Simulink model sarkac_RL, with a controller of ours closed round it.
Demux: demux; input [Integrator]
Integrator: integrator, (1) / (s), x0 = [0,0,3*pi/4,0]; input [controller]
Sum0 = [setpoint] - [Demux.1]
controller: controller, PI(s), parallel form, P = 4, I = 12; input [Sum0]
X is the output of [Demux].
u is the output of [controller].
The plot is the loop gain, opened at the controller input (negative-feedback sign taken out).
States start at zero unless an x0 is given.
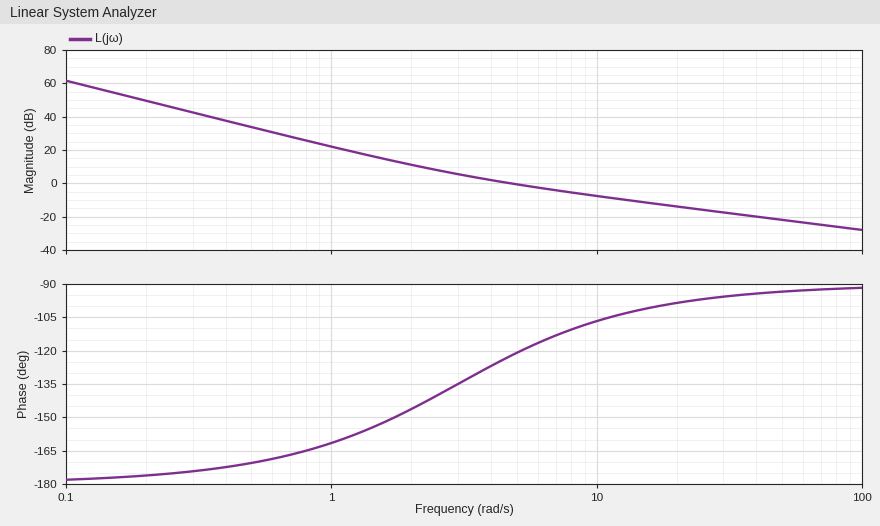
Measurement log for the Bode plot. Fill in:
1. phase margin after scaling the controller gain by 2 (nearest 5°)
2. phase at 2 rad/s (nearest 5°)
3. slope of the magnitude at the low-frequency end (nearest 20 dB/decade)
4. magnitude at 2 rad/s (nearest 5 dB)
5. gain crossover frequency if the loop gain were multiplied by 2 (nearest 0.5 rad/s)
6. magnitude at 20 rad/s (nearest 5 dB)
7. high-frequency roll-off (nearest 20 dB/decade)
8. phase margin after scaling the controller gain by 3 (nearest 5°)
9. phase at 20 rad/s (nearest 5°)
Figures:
70°
-145°
-40 dB/decade
10 dB
8.5 rad/s
-15 dB
-20 dB/decade
75°
-100°
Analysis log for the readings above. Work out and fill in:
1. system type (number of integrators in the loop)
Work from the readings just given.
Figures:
2
